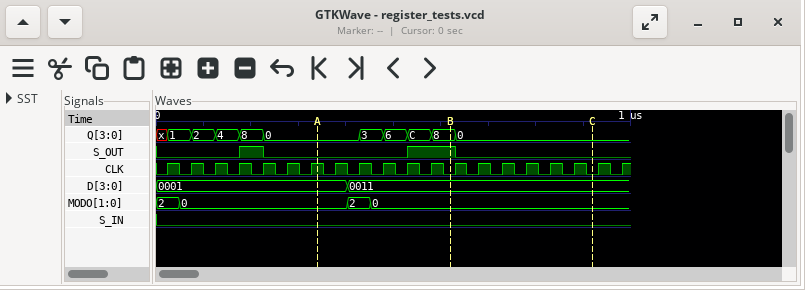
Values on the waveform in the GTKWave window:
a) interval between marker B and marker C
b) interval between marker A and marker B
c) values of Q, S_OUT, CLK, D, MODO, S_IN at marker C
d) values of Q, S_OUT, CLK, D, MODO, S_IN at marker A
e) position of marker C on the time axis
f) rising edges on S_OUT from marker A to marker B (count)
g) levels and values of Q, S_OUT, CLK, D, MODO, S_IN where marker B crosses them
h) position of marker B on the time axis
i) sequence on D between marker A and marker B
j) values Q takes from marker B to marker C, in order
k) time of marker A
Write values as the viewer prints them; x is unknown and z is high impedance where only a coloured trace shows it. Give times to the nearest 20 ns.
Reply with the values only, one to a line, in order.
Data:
300 ns
280 ns
Q=0, S_OUT=0, CLK=0, D=0011, MODO=0, S_IN=0
Q=0, S_OUT=0, CLK=1, D=0001, MODO=0, S_IN=0
920 ns
1
Q=8, S_OUT=1, CLK=0, D=0011, MODO=0, S_IN=0
620 ns
0001, 0011
8, 0
340 ns
